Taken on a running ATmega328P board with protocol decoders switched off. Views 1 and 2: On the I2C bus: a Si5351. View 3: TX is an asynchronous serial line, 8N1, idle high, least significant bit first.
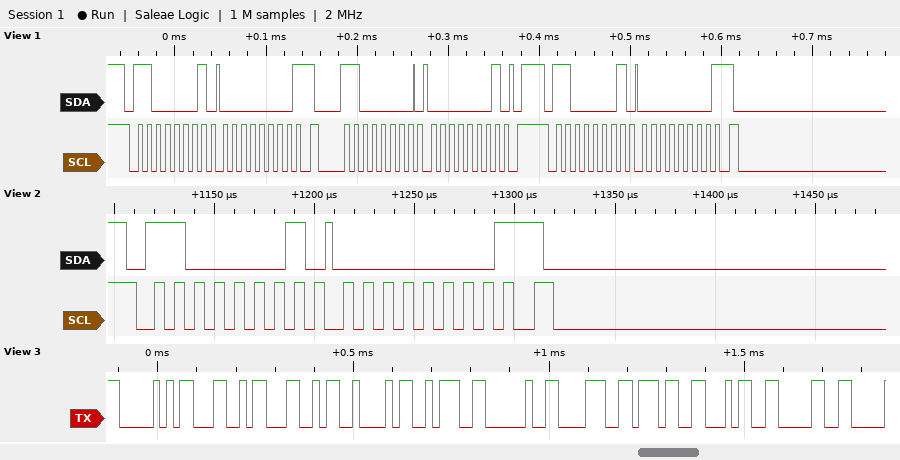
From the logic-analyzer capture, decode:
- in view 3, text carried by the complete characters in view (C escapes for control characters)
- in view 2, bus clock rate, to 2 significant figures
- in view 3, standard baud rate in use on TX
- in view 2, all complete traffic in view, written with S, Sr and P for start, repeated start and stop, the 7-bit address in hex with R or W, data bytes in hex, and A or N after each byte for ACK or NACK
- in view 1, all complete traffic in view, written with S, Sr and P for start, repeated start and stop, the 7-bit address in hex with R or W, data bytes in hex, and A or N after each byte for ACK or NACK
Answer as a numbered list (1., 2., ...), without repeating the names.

1. "PLLB: 8740"
2. 100 kHz
3. 57600 baud
4. S 60R A 00 N
5. S 60R A 00 N Sr 60W A 01 A P S 60R A 00 N
